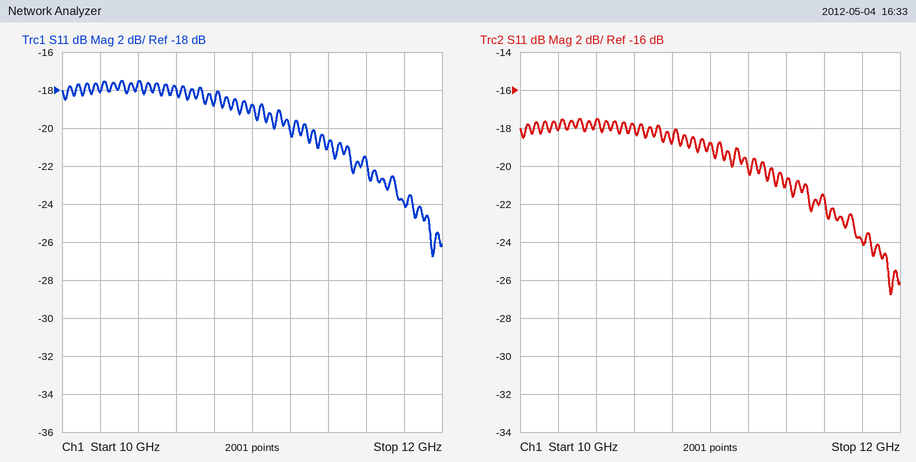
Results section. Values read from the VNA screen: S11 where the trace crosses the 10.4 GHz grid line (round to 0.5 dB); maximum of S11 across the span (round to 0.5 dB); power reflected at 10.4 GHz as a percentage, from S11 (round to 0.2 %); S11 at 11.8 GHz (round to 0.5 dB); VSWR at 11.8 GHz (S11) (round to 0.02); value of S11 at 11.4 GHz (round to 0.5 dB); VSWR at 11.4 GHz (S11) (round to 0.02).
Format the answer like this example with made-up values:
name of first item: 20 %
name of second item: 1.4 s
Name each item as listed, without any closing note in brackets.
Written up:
S11 where the trace crosses the 10.4 GHz grid line: -17.5 dB
maximum of S11 across the span: -17.5 dB
power reflected at 10.4 GHz as a percentage, from S11: 1.8 %
S11 at 11.8 GHz: -24.0 dB
VSWR at 11.8 GHz (S11): 1.14
value of S11 at 11.4 GHz: -21.0 dB
VSWR at 11.4 GHz (S11): 1.20
